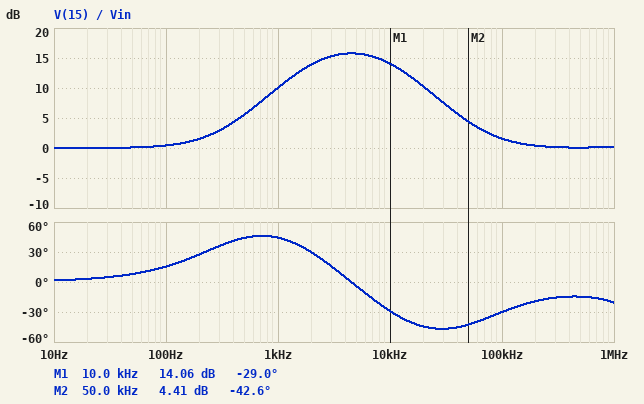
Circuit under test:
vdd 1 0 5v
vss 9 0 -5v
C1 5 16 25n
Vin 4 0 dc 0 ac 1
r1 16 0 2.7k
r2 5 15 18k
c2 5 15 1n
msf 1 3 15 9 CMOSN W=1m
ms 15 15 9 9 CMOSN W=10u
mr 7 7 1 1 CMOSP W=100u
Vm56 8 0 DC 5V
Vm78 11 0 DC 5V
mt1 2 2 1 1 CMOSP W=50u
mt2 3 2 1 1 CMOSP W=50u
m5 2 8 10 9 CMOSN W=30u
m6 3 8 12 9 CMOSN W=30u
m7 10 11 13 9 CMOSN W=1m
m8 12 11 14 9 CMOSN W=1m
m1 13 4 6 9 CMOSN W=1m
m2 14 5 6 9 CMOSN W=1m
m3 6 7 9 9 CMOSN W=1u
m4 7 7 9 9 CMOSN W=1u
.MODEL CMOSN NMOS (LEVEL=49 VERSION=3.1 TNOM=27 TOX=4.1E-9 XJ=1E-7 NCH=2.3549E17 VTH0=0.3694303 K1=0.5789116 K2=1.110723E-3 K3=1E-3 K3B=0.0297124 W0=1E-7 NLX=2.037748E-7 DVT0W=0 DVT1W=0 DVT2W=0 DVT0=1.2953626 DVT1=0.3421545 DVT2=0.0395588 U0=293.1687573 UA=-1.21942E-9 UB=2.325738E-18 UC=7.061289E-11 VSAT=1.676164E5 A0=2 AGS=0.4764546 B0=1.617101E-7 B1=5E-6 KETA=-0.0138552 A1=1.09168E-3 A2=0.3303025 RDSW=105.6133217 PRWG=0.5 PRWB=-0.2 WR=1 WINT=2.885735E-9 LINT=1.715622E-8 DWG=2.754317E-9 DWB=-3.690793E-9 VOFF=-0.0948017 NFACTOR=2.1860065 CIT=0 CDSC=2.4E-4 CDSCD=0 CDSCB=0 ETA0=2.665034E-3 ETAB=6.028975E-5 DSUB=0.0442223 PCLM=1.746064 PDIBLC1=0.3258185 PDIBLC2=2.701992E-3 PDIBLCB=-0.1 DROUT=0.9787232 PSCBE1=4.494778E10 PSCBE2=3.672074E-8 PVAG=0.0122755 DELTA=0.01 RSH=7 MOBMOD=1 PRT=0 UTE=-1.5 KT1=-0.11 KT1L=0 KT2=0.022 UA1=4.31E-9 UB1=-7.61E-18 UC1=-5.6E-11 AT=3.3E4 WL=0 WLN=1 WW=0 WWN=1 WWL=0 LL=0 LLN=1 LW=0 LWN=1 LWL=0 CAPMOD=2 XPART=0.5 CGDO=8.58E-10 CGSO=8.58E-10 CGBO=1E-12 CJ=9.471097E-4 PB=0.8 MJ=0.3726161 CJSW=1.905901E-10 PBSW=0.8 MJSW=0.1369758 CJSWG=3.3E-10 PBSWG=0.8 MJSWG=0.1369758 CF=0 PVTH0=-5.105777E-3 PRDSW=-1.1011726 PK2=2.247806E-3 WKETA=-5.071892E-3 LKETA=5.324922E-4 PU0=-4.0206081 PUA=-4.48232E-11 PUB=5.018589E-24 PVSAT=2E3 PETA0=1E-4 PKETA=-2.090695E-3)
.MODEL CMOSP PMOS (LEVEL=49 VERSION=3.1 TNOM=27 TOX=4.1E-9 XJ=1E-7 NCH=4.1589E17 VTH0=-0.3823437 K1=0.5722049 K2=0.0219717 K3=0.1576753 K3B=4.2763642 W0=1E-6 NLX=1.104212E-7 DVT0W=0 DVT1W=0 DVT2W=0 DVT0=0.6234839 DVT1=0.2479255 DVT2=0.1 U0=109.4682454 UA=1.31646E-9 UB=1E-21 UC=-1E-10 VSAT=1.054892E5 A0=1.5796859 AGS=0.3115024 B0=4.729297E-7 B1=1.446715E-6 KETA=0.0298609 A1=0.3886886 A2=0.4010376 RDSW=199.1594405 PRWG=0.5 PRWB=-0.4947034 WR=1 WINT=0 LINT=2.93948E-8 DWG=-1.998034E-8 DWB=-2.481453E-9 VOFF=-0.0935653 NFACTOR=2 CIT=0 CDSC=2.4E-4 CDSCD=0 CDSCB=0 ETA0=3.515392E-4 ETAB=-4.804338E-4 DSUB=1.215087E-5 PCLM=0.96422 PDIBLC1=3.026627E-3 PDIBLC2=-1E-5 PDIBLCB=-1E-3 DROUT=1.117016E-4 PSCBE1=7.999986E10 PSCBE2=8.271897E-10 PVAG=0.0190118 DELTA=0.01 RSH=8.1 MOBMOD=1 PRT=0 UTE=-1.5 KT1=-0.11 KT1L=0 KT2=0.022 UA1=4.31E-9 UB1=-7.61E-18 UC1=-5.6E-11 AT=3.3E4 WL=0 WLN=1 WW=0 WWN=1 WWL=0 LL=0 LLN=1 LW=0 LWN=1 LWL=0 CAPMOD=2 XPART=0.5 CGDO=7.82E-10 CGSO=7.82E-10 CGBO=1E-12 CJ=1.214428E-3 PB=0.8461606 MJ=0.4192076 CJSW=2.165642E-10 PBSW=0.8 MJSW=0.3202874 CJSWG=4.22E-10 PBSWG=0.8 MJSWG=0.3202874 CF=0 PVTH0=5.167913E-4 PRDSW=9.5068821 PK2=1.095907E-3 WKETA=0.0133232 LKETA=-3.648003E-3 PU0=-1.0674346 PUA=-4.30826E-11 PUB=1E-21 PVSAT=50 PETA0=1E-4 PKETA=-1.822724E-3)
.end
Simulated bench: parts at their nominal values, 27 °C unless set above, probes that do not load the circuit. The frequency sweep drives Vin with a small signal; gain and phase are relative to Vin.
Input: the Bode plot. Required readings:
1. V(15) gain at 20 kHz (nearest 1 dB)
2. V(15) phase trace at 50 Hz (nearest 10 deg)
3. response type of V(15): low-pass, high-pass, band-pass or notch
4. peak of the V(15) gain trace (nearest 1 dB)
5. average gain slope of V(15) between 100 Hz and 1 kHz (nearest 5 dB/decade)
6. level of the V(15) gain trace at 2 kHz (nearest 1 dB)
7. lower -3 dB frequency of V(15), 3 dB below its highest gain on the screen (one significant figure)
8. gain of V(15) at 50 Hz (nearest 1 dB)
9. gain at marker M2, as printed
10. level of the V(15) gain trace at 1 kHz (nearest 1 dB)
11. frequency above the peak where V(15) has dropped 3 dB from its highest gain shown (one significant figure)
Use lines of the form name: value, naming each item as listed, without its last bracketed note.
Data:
V(15) gain at 20 kHz: 10 dB
V(15) phase trace at 50 Hz: 10 deg
response type of V(15): low-pass, high-pass, band-pass or notch: band-pass
peak of the V(15) gain trace: 16 dB
average gain slope of V(15) between 100 Hz and 1 kHz: 10 dB/decade
level of the V(15) gain trace at 2 kHz: 14 dB
lower -3 dB frequency of V(15), 3 dB below its highest gain on the screen: 2 kHz
gain of V(15) at 50 Hz: 0 dB
gain at marker M2, as printed: 4.41 dB
level of the V(15) gain trace at 1 kHz: 10 dB
frequency above the peak where V(15) has dropped 3 dB from its highest gain shown: 10 kHz
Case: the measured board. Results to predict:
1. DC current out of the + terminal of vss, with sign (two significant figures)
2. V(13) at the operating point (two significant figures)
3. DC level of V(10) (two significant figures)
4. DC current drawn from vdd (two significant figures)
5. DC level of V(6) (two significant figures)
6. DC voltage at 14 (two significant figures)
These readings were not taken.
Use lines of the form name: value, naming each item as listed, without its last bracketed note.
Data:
DC current out of the + terminal of vss, with sign: -3.0 mA
V(13) at the operating point: 3.1 V
DC level of V(10): 3.1 V
DC current drawn from vdd: 3.0 mA
DC level of V(6): -1.1 V
DC voltage at 14: 1.5 V
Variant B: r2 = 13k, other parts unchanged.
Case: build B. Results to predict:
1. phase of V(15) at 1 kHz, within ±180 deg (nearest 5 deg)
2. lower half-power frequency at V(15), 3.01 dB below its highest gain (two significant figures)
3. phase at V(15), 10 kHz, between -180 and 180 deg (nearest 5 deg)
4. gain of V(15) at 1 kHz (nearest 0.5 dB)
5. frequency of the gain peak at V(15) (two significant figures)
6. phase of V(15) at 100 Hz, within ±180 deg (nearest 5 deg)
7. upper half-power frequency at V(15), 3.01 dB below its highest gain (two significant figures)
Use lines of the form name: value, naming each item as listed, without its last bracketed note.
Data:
phase of V(15) at 1 kHz, within ±180 deg: 40 deg
lower half-power frequency at V(15), 3.01 dB below its highest gain: 1.7 kHz
phase at V(15), 10 kHz, between -180 and 180 deg: -20 deg
gain of V(15) at 1 kHz: 8.0 dB
frequency of the gain peak at V(15): 5.3 kHz
phase of V(15) at 100 Hz, within ±180 deg: 10 deg
upper half-power frequency at V(15), 3.01 dB below its highest gain: 17 kHz
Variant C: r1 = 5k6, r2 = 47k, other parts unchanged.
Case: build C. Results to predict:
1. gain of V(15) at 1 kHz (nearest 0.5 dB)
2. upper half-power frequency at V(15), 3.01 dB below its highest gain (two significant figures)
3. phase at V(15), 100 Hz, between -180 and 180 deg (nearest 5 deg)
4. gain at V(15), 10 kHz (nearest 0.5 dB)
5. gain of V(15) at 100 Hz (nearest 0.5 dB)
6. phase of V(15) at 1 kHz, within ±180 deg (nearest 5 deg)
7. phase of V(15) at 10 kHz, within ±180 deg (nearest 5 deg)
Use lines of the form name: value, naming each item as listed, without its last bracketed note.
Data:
gain of V(15) at 1 kHz: 15.5 dB
upper half-power frequency at V(15), 3.01 dB below its highest gain: 5.4 kHz
phase at V(15), 100 Hz, between -180 and 180 deg: 35 deg
gain at V(15), 10 kHz: 10.0 dB
gain of V(15) at 100 Hz: 2.5 dB
phase of V(15) at 1 kHz, within ±180 deg: 25 deg
phase of V(15) at 10 kHz, within ±180 deg: -50 deg
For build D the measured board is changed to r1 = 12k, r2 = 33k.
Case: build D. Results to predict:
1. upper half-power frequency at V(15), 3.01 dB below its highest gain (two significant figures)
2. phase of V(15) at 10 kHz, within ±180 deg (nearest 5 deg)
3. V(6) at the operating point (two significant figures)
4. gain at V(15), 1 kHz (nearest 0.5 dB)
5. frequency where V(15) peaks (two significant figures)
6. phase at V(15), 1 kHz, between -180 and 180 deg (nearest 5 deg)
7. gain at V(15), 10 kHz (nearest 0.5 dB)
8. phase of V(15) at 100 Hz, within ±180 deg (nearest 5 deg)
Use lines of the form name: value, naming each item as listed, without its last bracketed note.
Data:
upper half-power frequency at V(15), 3.01 dB below its highest gain: 6.3 kHz
phase of V(15) at 10 kHz, within ±180 deg: -35 deg
V(6) at the operating point: -1.1 V
gain at V(15), 1 kHz: 10.5 dB
frequency where V(15) peaks: 1.6 kHz
phase at V(15), 1 kHz, between -180 and 180 deg: 10 deg
gain at V(15), 10 kHz: 5.5 dB
phase of V(15) at 100 Hz, within ±180 deg: 25 deg
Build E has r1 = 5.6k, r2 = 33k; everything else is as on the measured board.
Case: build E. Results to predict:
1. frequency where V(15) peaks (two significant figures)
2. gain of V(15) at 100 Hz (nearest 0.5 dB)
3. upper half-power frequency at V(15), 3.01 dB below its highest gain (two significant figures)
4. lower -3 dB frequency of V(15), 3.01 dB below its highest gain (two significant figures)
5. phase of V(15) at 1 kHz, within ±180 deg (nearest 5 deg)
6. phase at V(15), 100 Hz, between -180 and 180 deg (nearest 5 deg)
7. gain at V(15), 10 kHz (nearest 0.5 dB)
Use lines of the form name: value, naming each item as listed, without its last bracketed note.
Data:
frequency where V(15) peaks: 2.3 kHz
gain of V(15) at 100 Hz: 1.5 dB
upper half-power frequency at V(15), 3.01 dB below its highest gain: 7.0 kHz
lower -3 dB frequency of V(15), 3.01 dB below its highest gain: 780 Hz
phase of V(15) at 1 kHz, within ±180 deg: 30 deg
phase at V(15), 100 Hz, between -180 and 180 deg: 25 deg
gain at V(15), 10 kHz: 10.0 dB
